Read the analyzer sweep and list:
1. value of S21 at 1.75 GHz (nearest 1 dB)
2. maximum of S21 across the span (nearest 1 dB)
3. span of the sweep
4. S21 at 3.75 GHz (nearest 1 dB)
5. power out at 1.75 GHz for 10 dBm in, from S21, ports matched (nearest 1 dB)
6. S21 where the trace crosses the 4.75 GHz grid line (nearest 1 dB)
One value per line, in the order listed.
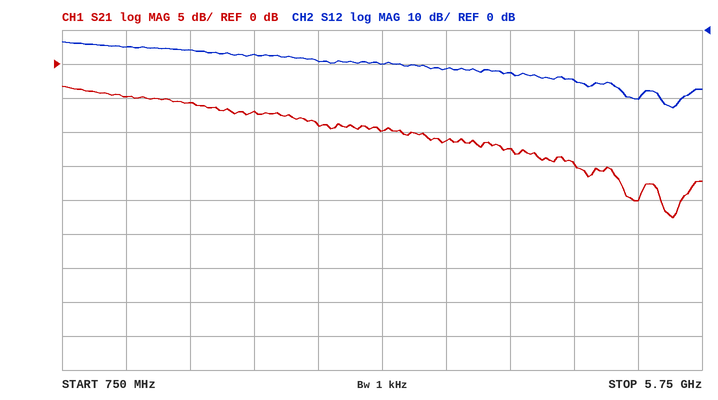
-6 dB
-3 dB
5 GHz
-11 dB
4 dBm
-15 dB
